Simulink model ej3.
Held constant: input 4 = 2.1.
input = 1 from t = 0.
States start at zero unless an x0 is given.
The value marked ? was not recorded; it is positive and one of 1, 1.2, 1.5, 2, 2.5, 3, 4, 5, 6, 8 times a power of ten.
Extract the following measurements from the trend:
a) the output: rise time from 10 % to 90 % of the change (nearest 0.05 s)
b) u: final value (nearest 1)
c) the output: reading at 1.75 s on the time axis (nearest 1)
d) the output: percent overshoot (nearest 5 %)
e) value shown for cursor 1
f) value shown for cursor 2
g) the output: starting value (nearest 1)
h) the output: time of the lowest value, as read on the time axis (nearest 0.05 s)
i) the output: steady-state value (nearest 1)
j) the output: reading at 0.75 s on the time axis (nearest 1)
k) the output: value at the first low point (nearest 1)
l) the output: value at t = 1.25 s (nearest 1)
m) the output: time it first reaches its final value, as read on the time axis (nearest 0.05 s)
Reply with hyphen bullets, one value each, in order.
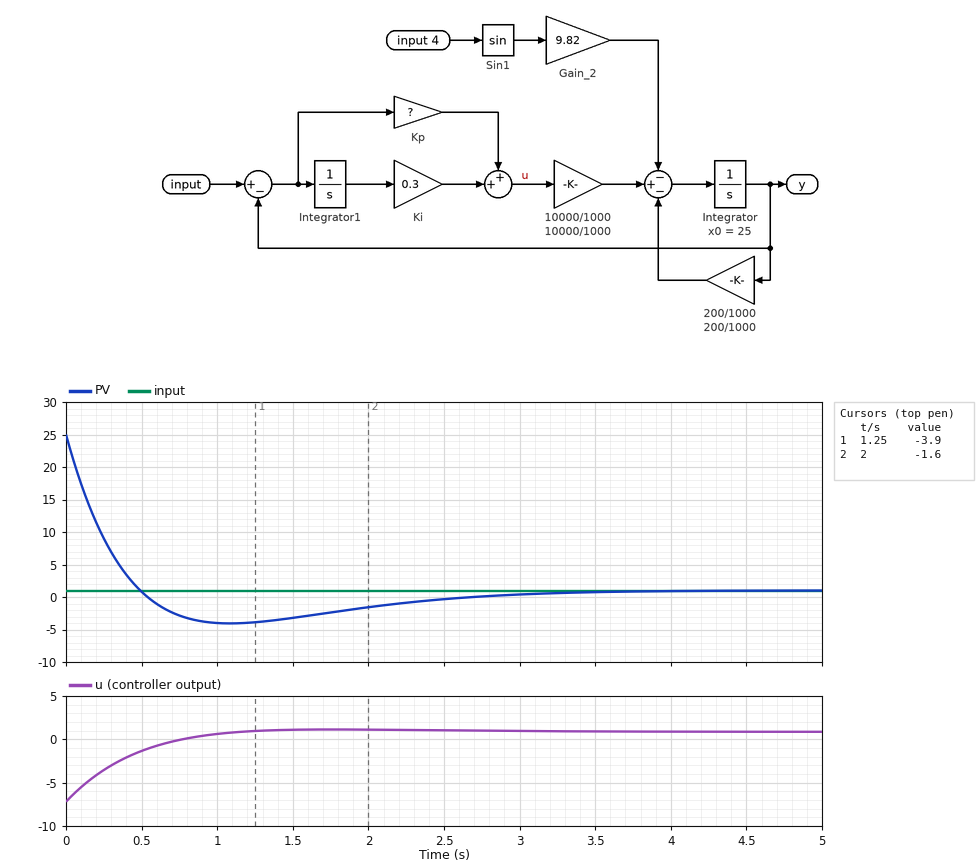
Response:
- 0.35 s
- 1
- -2
- 20 %
- -3.9
- -1.6
- 25
- 1.10 s
- 1
- -3
- -4
- -4
- 0.50 s
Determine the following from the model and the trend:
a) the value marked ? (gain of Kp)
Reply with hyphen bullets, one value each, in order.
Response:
- 0.3
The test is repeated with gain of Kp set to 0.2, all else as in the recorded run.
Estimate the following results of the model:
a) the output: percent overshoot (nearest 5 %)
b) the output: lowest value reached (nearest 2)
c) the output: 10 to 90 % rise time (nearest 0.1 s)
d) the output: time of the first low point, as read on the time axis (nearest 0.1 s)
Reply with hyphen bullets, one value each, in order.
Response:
- 30 %
- -6
- 0.4 s
- 1.2 s
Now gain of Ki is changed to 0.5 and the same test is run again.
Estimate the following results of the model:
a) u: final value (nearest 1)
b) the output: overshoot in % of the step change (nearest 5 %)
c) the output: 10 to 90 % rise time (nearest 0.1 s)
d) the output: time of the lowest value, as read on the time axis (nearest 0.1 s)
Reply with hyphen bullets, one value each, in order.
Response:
- 1
- 25 %
- 0.3 s
- 0.9 s
